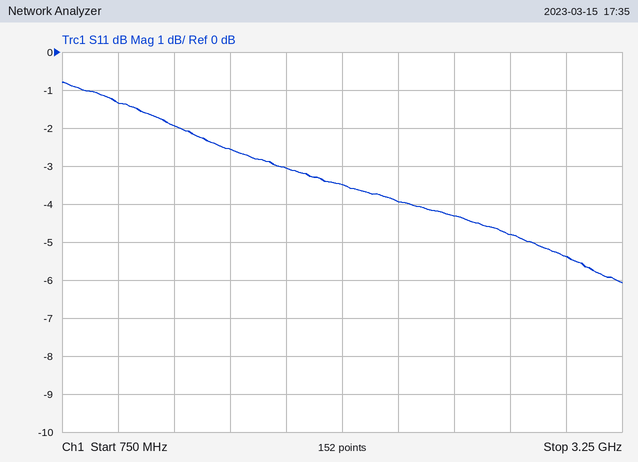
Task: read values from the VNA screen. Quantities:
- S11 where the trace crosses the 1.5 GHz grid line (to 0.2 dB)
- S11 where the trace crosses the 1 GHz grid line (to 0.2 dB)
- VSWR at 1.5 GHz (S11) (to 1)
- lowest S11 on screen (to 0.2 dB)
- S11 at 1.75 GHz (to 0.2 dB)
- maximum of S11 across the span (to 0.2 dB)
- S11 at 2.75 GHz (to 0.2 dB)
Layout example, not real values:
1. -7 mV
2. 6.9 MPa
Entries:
1. -2.6 dB
2. -1.4 dB
3. 7
4. -6.0 dB
5. -3.0 dB
6. -0.8 dB
7. -4.8 dB
